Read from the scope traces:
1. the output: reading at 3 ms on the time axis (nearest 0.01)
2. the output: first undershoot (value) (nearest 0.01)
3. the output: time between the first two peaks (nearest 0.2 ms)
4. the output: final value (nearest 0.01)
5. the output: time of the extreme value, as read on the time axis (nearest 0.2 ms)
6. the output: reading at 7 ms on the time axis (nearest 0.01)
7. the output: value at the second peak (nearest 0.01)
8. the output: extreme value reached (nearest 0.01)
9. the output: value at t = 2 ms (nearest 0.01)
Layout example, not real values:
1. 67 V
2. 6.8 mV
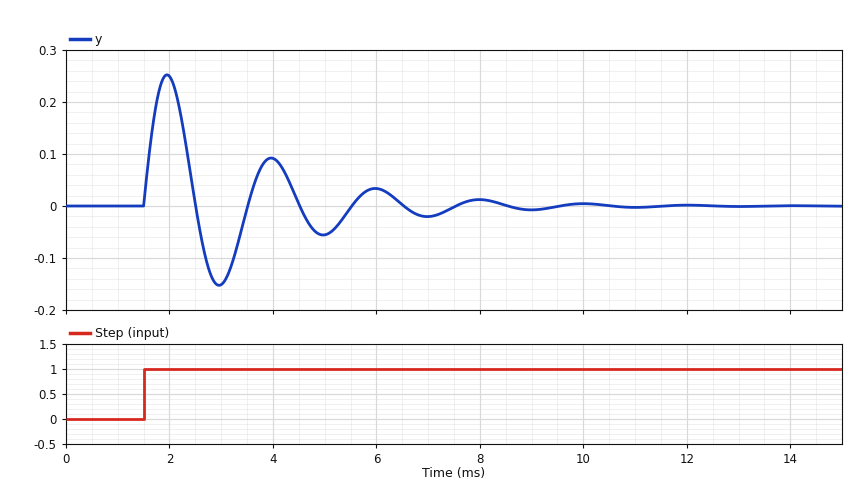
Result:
1. -0.15
2. -0.15
3. 2.0 ms
4. 0.00
5. 2.0 ms
6. -0.02
7. 0.09
8. 0.25
9. 0.25
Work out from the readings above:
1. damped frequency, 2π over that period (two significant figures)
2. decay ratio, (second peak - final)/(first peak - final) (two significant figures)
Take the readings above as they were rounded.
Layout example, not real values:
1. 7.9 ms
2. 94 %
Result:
1. 3.1 rad/ms
2. 0.36
